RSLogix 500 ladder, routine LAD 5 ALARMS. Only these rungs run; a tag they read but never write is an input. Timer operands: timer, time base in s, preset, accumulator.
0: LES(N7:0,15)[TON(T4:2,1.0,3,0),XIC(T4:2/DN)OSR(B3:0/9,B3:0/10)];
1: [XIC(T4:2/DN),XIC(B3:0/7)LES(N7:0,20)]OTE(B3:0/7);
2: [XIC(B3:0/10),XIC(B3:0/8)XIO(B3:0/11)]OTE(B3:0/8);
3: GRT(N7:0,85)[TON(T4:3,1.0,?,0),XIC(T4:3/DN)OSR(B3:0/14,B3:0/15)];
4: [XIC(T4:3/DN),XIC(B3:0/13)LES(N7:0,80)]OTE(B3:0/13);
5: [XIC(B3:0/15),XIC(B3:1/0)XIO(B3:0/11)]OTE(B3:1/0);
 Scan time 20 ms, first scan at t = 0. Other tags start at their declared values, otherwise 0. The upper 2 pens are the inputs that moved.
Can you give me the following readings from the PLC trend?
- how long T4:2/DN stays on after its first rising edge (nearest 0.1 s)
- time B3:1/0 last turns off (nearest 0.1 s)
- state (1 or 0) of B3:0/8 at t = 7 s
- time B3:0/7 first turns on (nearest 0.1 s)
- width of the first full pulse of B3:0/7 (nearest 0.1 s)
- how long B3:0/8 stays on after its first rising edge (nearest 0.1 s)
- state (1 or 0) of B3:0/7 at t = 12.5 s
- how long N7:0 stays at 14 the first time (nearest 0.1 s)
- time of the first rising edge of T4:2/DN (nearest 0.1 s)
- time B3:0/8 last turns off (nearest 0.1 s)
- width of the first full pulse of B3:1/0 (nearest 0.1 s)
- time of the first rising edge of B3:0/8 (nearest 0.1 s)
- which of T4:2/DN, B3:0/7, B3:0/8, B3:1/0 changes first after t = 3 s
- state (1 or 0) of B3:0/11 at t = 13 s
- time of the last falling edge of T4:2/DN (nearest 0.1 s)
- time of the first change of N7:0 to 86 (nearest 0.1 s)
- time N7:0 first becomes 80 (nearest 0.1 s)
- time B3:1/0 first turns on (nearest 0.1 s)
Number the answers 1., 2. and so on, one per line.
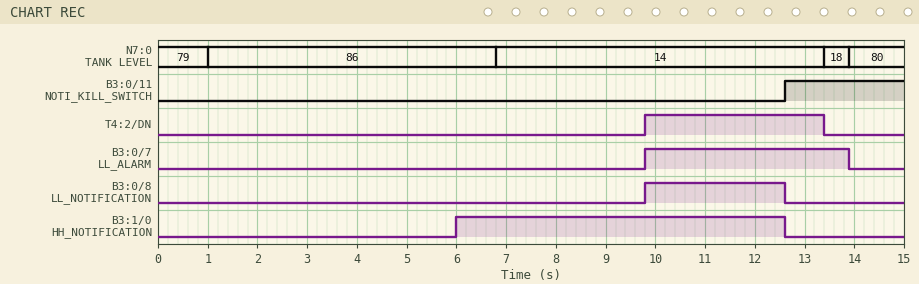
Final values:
1. 3.6 s
2. 12.6 s
3. 0
4. 9.8 s
5. 4.1 s
6. 2.8 s
7. 1
8. 6.6 s
9. 9.8 s
10. 12.6 s
11. 6.6 s
12. 9.8 s
13. B3:1/0
14. 1
15. 13.4 s
16. 1.0 s
17. 13.9 s
18. 6.0 s
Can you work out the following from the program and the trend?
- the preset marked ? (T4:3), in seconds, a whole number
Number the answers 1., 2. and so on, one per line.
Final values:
1. 5 s
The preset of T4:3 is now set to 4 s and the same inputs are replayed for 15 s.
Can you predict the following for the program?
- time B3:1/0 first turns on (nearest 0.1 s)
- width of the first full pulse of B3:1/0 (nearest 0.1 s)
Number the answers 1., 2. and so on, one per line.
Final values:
1. 5.0 s
2. 7.6 s
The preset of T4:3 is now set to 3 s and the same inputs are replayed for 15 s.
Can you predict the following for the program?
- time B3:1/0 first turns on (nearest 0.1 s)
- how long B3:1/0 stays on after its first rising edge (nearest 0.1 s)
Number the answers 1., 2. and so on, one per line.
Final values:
1. 4.0 s
2. 8.6 s
